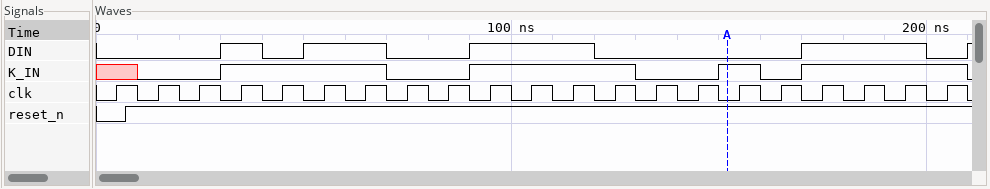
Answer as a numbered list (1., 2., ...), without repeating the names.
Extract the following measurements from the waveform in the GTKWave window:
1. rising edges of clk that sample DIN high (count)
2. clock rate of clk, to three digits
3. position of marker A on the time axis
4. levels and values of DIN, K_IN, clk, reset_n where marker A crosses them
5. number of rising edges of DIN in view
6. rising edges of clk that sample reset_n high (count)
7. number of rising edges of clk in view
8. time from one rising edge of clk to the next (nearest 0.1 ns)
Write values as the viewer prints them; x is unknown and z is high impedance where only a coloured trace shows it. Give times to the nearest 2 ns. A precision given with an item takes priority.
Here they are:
1. 9
2. 100 MHz
3. 152 ns
4. DIN=0, K_IN=1, clk=0, reset_n=1
5. 5
6. 20
7. 21
8. 10 ns
